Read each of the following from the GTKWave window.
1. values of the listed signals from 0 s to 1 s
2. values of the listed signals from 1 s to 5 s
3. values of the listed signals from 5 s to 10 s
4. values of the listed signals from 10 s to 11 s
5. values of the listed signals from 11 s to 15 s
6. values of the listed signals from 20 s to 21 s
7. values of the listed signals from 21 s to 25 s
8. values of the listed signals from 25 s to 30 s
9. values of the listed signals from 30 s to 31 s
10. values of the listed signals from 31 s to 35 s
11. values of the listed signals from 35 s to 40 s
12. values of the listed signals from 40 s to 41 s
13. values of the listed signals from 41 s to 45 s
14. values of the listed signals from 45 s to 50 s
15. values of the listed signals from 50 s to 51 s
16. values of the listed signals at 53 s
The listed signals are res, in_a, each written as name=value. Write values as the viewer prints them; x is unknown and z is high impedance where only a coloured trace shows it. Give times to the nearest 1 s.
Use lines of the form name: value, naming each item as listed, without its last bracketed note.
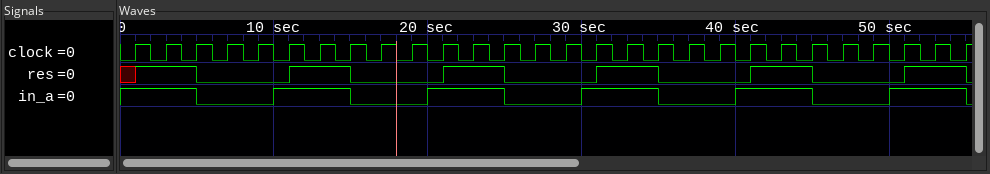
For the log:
values of the listed signals from 0 s to 1 s: res=x, in_a=1
values of the listed signals from 1 s to 5 s: res=1, in_a=1
values of the listed signals from 5 s to 10 s: res=0, in_a=0
values of the listed signals from 10 s to 11 s: res=0, in_a=1
values of the listed signals from 11 s to 15 s: res=1, in_a=1
values of the listed signals from 20 s to 21 s: res=0, in_a=1
values of the listed signals from 21 s to 25 s: res=1, in_a=1
values of the listed signals from 25 s to 30 s: res=0, in_a=0
values of the listed signals from 30 s to 31 s: res=0, in_a=1
values of the listed signals from 31 s to 35 s: res=1, in_a=1
values of the listed signals from 35 s to 40 s: res=0, in_a=0
values of the listed signals from 40 s to 41 s: res=0, in_a=1
values of the listed signals from 41 s to 45 s: res=1, in_a=1
values of the listed signals from 45 s to 50 s: res=0, in_a=0
values of the listed signals from 50 s to 51 s: res=0, in_a=1
values of the listed signals at 53 s: res=1, in_a=1
